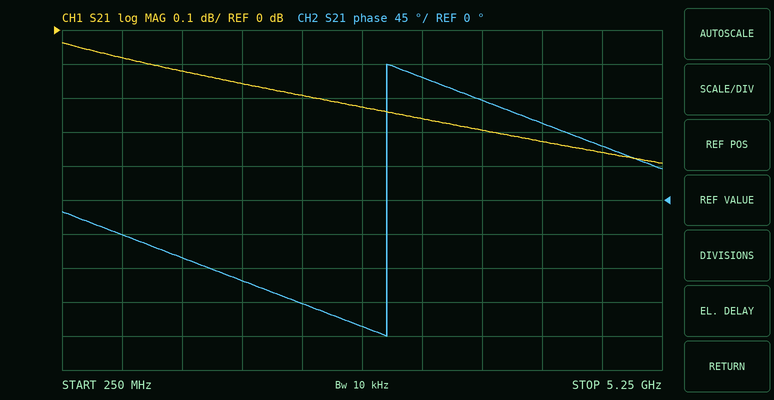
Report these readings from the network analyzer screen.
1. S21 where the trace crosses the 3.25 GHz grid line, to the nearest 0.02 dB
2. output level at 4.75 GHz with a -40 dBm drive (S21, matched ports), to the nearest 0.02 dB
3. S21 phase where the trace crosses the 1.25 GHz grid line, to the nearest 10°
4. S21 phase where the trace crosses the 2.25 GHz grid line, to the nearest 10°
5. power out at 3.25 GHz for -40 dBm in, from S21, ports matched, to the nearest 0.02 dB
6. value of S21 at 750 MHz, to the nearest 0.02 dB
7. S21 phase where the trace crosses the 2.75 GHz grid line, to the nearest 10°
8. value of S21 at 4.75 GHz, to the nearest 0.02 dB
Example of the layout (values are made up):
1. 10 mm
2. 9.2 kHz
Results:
1. -0.26 dB
2. -40.36 dBm
3. -80°
4. -140°
5. -40.26 dBm
6. -0.08 dB
7. -170°
8. -0.36 dB
